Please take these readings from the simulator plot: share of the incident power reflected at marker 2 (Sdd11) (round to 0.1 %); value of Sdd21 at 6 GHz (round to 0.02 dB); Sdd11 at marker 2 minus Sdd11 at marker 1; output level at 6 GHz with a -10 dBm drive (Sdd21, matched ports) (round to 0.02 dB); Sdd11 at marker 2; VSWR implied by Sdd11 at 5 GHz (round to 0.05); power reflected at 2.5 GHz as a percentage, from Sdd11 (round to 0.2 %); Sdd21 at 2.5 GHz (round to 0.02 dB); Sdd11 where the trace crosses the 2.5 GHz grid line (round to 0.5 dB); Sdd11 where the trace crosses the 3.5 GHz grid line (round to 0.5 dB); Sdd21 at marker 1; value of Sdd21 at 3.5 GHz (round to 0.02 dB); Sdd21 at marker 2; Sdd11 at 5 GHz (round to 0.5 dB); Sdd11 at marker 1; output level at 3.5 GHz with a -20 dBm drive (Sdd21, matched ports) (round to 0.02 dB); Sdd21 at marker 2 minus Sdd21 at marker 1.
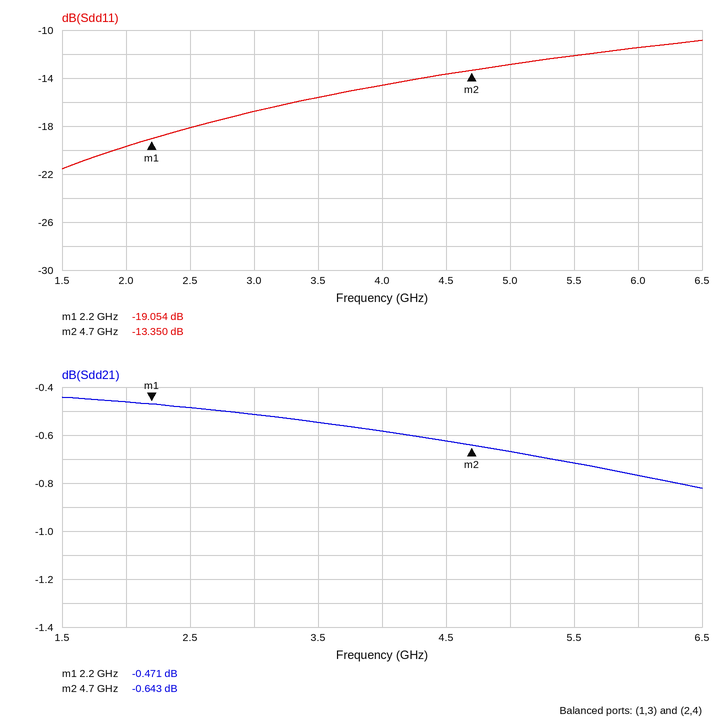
4.6 %
-0.76 dB
5.704 dB
-10.76 dBm
-13.350 dB
1.60
1.6 %
-0.48 dB
-18.0 dB
-15.5 dB
-0.471 dB
-0.54 dB
-0.643 dB
-13.0 dB
-19.054 dB
-20.54 dBm
-0.172 dB
